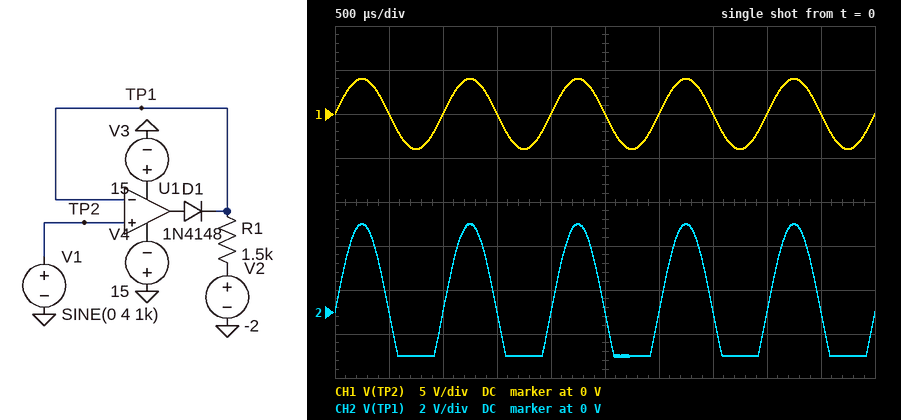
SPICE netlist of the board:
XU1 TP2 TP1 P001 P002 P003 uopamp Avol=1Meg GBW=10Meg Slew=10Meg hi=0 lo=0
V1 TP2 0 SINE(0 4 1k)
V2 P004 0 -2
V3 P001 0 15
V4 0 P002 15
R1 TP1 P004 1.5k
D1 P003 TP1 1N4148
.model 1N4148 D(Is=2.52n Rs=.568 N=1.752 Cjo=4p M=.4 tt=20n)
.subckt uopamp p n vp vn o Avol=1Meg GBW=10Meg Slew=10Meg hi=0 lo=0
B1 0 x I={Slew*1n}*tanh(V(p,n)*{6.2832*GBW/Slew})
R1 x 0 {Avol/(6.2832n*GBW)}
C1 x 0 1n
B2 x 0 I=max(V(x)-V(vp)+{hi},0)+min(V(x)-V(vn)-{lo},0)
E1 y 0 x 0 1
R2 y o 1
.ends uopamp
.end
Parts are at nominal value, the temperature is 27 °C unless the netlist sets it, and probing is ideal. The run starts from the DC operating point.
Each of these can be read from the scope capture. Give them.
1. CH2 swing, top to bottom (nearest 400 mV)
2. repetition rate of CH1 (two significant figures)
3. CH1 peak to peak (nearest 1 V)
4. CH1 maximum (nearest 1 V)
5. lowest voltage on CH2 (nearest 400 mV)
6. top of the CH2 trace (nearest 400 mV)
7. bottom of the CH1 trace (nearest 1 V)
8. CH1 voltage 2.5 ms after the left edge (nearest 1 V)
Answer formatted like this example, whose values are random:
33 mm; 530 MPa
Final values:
6.0 V; 1.0 kHz; 8 V; 4 V; -2.0 V; 4.0 V; -4 V; 0 V
